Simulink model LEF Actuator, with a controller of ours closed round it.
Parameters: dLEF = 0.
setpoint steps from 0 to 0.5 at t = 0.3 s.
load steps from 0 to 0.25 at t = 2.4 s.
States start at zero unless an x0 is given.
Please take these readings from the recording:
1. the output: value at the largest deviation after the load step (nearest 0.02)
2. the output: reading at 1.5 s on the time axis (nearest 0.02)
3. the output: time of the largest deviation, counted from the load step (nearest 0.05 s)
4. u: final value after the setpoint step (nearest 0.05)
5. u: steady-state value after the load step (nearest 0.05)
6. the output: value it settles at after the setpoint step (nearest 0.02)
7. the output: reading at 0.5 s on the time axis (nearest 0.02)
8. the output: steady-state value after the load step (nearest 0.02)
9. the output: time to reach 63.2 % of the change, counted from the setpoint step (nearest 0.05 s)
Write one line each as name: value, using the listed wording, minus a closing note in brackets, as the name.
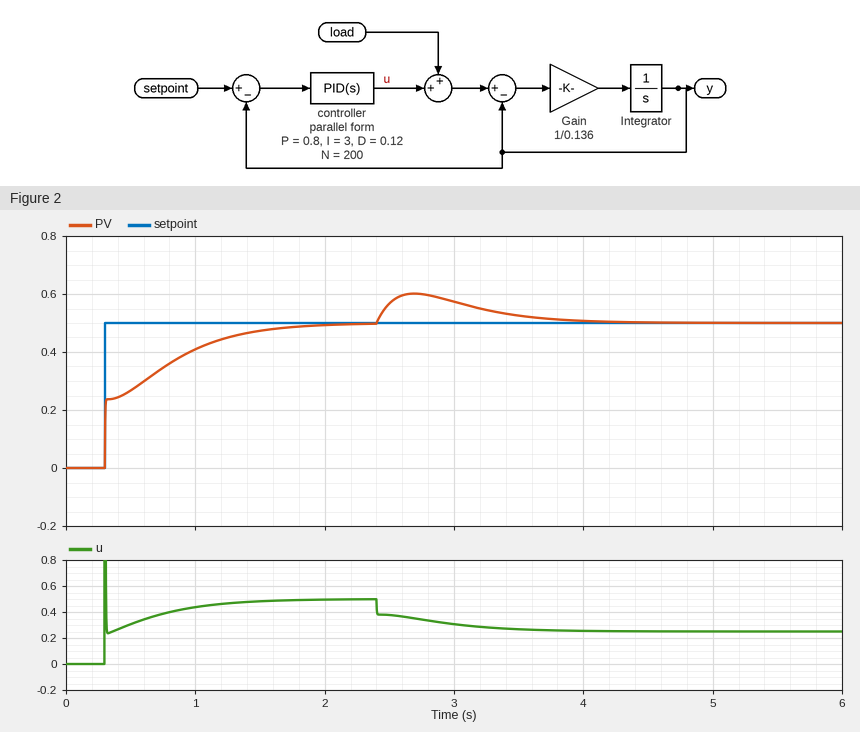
the output: value at the largest deviation after the load step: 0.60
the output: reading at 1.5 s on the time axis: 0.48
the output: time of the largest deviation, counted from the load step: 0.30 s
u: final value after the setpoint step: 0.50
u: steady-state value after the load step: 0.25
the output: value it settles at after the setpoint step: 0.50
the output: reading at 0.5 s on the time axis: 0.26
the output: steady-state value after the load step: 0.50
the output: time to reach 63.2 % of the change, counted from the setpoint step: 0.35 s
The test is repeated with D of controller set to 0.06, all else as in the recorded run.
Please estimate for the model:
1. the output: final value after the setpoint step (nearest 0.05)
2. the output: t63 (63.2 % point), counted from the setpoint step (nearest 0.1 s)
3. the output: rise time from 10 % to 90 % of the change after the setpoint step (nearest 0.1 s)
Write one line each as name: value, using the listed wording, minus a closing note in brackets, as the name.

the output: final value after the setpoint step: 0.50
the output: t63 (63.2 % point), counted from the setpoint step: 0.3 s
the output: rise time from 10 % to 90 % of the change after the setpoint step: 0.9 s
